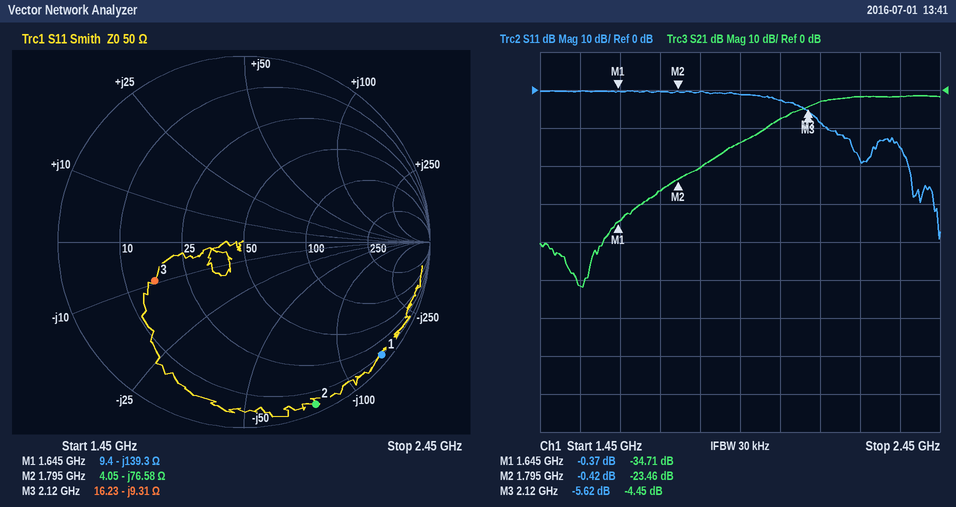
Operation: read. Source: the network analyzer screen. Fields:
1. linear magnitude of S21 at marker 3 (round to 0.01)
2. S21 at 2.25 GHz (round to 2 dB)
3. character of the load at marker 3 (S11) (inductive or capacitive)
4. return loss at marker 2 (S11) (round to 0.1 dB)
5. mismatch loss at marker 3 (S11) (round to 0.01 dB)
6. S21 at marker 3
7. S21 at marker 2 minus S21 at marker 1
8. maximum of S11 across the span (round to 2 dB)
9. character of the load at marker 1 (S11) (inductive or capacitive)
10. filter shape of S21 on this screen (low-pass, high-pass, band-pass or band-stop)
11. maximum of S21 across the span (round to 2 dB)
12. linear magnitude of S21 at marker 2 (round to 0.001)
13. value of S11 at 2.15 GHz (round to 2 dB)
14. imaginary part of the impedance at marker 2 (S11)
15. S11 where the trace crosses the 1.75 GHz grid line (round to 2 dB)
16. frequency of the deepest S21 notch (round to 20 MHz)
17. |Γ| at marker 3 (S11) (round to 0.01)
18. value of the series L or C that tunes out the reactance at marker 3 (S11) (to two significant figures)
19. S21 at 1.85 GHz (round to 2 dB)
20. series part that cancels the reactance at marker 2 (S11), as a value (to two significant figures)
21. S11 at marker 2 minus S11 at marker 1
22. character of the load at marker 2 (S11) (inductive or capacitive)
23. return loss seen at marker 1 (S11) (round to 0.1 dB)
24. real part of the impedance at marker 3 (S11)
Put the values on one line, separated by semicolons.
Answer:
0.60; -2 dB; capacitive; 0.4 dB; 1.39 dB; -4.45 dB; 11.25 dB; 0 dB; capacitive; high-pass; -2 dB; 0.067; -8 dB; -76.58 Ω; 0 dB; 1.56 GHz; 0.52; 700 pH; -20 dB; 6.8 nH; -0.05 dB; capacitive; 0.4 dB; 16.23 Ω
